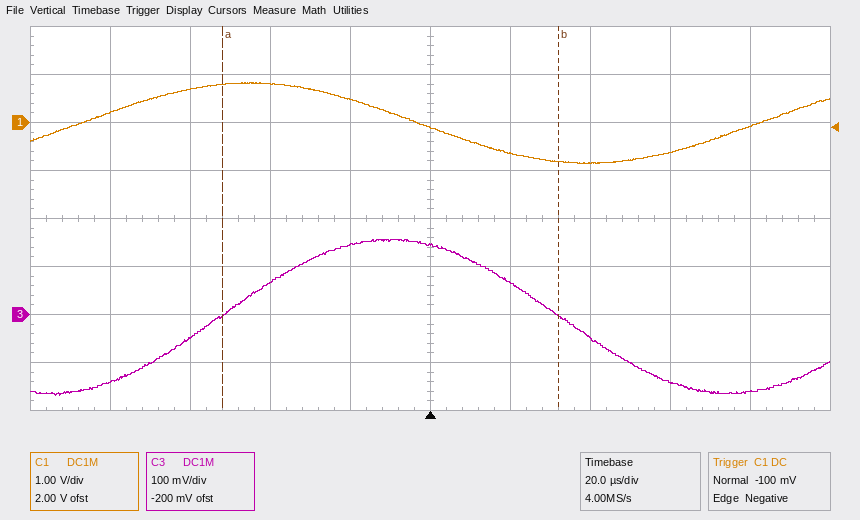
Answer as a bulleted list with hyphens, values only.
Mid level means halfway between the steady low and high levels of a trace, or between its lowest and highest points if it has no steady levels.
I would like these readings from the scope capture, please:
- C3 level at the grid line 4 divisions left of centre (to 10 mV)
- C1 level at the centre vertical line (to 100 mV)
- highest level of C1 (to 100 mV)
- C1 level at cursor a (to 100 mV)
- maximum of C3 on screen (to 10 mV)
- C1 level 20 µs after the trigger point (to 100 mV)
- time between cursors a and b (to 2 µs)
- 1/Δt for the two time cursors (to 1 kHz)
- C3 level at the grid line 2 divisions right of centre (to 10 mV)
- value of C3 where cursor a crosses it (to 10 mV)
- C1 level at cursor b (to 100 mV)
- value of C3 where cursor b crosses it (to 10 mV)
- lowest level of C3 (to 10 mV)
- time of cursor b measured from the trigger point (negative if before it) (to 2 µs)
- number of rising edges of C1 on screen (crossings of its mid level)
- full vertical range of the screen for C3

- -140 mV
- -100 mV
- 800 mV
- 800 mV
- 160 mV
- -600 mV
- 84 µs
- 12 kHz
- -50 mV
- 0 mV
- -800 mV
- 0 mV
- -170 mV
- +32 µs
- 2
- 800 mV
